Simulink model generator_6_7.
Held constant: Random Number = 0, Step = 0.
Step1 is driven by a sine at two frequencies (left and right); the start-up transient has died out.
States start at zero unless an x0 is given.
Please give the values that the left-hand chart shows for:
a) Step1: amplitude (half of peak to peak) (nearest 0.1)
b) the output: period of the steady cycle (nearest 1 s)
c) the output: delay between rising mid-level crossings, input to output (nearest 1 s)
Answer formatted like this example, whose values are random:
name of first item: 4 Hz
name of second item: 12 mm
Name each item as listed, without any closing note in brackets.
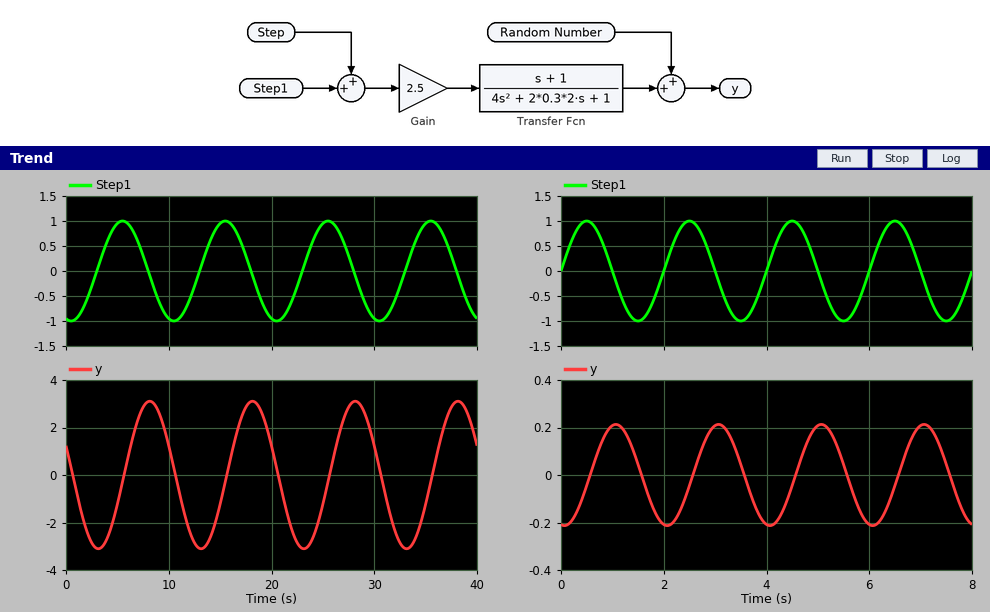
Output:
Step1: amplitude (half of peak to peak): 1.0
the output: period of the steady cycle: 10 s
the output: delay between rising mid-level crossings, input to output: 3 s
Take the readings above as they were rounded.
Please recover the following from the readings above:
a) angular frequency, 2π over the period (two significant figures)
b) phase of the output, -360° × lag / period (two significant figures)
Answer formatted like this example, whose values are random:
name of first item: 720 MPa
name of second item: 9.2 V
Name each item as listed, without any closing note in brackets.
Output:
angular frequency, 2π over the period: 0.63 rad/s
phase of the output, -360° × lag / period: -110°
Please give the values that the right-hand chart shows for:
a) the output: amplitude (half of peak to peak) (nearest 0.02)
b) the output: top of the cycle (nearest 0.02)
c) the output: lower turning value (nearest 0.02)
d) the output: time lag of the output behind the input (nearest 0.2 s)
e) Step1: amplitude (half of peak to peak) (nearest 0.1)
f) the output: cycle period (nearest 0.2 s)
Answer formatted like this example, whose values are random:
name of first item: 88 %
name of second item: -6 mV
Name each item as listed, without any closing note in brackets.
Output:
the output: amplitude (half of peak to peak): 0.22
the output: top of the cycle: 0.22
the output: lower turning value: -0.22
the output: time lag of the output behind the input: 0.6 s
Step1: amplitude (half of peak to peak): 1.0
the output: cycle period: 2.0 s
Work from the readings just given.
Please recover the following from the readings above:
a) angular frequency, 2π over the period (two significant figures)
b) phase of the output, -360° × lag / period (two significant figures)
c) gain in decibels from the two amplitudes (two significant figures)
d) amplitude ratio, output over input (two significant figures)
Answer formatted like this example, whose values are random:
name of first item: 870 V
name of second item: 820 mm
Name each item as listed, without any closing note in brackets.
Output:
angular frequency, 2π over the period: 3.1 rad/s
phase of the output, -360° × lag / period: -110°
gain in decibels from the two amplitudes: -13 dB
amplitude ratio, output over input: 0.22
